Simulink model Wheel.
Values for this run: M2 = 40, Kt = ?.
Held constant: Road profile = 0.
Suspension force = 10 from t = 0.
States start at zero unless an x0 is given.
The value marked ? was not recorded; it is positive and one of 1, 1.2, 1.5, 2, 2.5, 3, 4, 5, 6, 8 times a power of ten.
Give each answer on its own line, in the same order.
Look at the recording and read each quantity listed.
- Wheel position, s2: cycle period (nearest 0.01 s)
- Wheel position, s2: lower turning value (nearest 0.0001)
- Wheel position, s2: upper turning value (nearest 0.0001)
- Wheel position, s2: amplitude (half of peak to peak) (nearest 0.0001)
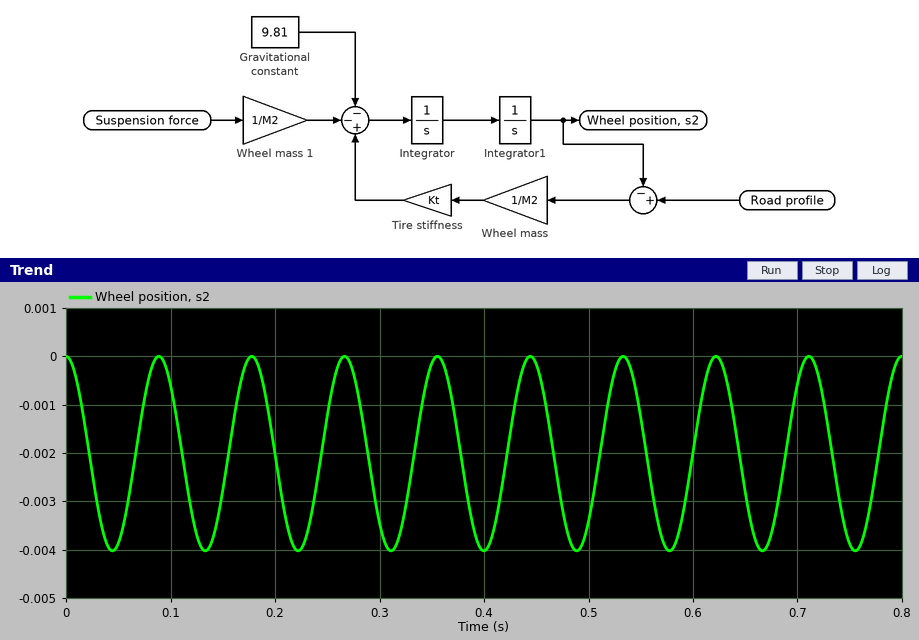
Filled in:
0.09 s
-0.0040
0.0000
0.0020
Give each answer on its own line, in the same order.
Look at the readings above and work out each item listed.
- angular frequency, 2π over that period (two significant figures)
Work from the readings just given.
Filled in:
70 rad/s
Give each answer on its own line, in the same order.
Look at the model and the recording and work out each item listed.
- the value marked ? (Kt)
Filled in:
200000
